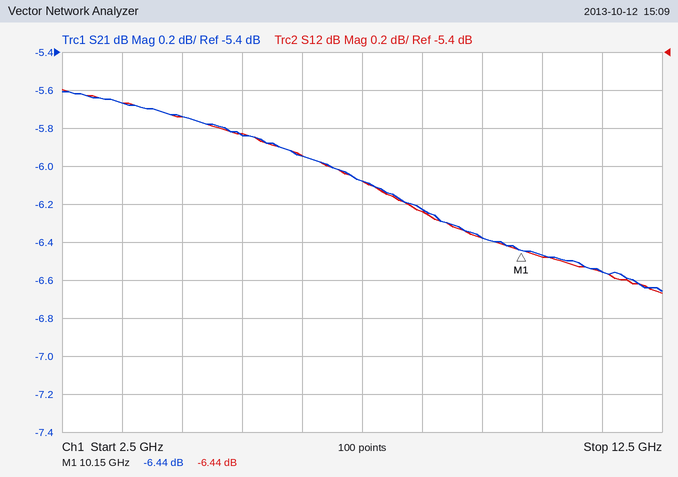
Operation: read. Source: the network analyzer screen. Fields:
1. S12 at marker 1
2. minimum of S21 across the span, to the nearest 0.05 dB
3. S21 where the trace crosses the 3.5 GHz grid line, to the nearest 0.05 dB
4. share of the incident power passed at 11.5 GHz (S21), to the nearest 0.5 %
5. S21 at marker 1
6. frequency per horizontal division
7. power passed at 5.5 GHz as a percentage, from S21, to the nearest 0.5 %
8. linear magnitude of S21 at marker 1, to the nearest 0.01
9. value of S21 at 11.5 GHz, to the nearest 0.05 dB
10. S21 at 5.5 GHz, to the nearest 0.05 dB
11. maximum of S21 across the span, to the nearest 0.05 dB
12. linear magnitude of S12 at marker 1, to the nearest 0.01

-6.44 dB
-6.65 dB
-5.65 dB
22.0 %
-6.44 dB
1 GHz
26.0 %
0.48
-6.55 dB
-5.85 dB
-5.60 dB
0.48
